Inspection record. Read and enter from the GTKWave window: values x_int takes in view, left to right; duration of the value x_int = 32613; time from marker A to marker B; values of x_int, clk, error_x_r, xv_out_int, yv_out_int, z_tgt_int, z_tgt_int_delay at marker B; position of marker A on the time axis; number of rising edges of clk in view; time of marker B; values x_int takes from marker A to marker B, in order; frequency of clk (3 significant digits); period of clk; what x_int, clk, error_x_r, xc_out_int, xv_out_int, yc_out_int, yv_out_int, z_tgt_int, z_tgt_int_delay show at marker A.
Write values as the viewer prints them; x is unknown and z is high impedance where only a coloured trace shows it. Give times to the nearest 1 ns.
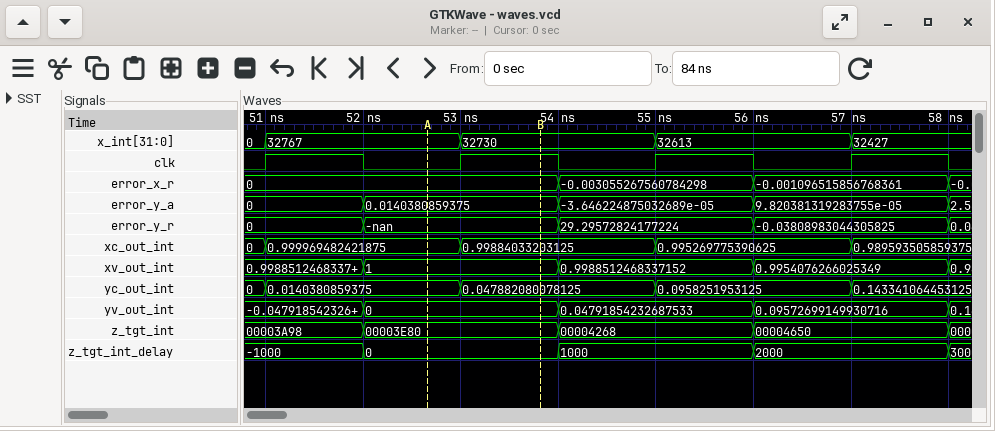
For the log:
0, 32767, 32730, 32613, 32427
2 ns
1 ns
x_int=32730, clk=1, error_x_r=0, xv_out_int=1, yv_out_int=0, z_tgt_int=00003E80, z_tgt_int_delay=0
53 ns
4
54 ns
32767, 32730
500 MHz
2 ns
x_int=32767, clk=0, error_x_r=0, xc_out_int=0.999969482421875, xv_out_int=1, yc_out_int=0.0140380859375, yv_out_int=0, z_tgt_int=00003E80, z_tgt_int_delay=0
